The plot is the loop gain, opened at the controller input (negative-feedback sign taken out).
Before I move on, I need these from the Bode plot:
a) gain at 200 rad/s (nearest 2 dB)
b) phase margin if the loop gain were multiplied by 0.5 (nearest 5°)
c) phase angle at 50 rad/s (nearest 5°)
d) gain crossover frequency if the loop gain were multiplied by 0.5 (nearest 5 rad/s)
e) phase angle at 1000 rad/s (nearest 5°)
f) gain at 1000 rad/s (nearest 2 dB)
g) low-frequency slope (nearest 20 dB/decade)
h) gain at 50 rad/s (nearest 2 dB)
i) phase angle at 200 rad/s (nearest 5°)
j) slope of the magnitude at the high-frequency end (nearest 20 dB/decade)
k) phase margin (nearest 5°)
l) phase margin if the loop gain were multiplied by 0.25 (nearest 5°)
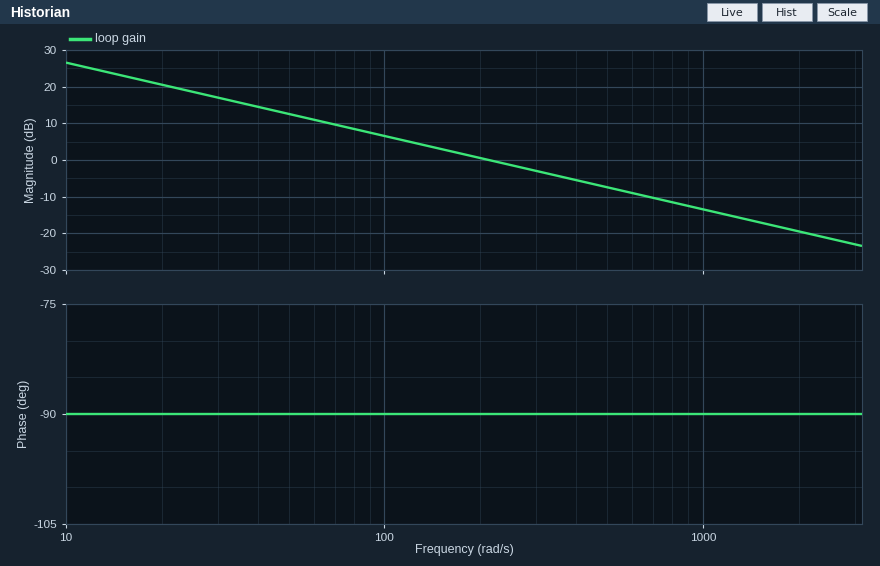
0 dB
90°
-90°
105 rad/s
-90°
-14 dB
-20 dB/decade
12 dB
-90°
-20 dB/decade
90°
90°
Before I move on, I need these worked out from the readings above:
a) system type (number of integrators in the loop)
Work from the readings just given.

1
